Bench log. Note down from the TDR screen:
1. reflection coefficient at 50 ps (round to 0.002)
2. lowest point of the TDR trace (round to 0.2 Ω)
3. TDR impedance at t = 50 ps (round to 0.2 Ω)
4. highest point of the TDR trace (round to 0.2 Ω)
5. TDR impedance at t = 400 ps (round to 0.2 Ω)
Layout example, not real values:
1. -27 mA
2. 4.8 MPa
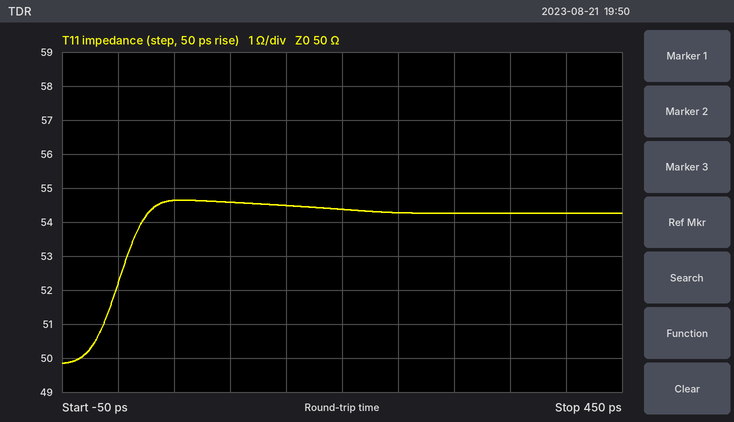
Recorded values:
1. +0.044
2. 49.8 Ω
3. 54.6 Ω
4. 54.6 Ω
5. 54.2 Ω
